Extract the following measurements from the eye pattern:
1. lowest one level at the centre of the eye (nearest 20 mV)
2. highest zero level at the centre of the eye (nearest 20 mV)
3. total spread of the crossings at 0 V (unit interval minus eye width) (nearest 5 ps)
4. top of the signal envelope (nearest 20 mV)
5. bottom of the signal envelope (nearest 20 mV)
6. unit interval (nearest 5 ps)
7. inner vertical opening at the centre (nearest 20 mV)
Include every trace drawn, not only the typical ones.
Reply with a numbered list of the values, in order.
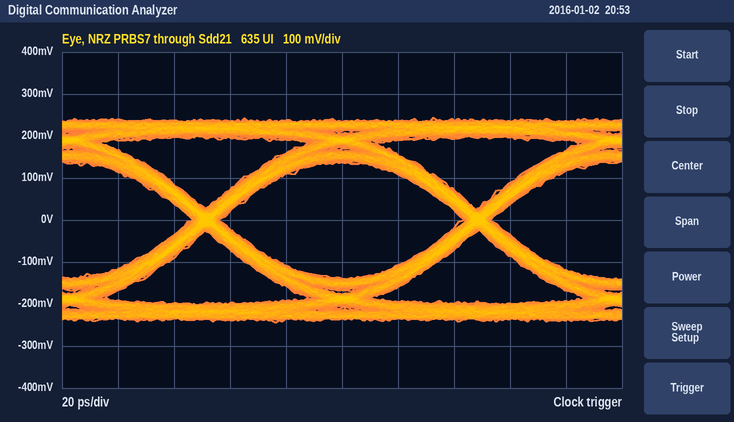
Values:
1. 140 mV
2. -140 mV
3. 10 ps
4. 240 mV
5. -240 mV
6. 95 ps
7. 280 mV
